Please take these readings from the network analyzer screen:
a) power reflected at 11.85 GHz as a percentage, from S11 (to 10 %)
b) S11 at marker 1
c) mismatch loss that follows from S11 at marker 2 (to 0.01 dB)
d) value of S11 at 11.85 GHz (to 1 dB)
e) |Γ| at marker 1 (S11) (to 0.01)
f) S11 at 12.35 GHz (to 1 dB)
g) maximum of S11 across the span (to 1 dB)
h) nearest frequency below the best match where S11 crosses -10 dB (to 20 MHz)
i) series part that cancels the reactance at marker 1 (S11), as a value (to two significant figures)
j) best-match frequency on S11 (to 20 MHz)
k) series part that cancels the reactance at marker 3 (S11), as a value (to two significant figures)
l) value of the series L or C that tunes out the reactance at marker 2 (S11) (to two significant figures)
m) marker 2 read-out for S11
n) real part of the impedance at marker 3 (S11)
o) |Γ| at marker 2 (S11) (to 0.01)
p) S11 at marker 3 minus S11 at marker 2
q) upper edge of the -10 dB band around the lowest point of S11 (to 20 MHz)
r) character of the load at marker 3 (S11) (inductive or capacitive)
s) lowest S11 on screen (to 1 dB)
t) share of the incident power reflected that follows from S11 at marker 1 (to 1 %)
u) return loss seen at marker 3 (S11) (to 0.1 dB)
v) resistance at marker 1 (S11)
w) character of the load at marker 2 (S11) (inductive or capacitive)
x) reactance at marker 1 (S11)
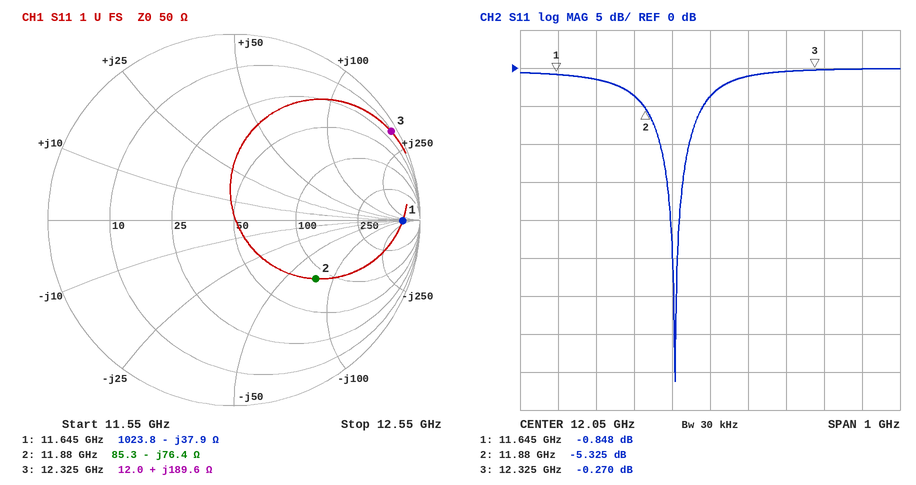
40 %
-0.848 dB
1.51 dB
-4 dB
0.91
0 dB
0 dB
11.92 GHz
520 pH
11.96 GHz
68 fF
1.0 nH
-5.325 dB
12.0 Ω
0.54
5.055 dB
12.00 GHz
inductive
-41 dB
82 %
0.3 dB
1023.8 Ω
capacitive
-37.9 Ω
